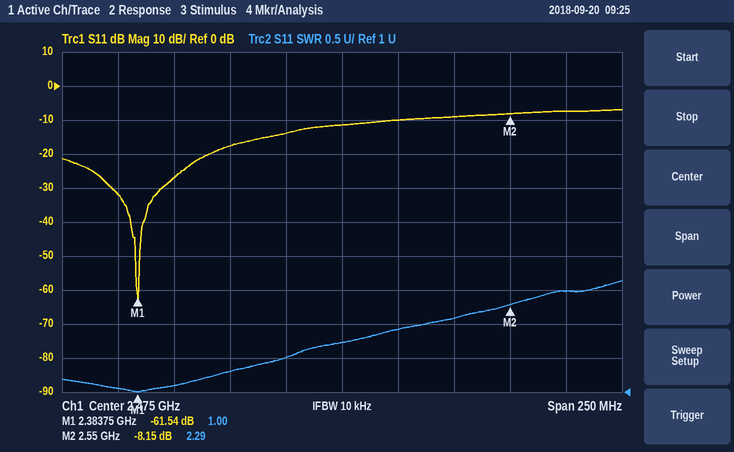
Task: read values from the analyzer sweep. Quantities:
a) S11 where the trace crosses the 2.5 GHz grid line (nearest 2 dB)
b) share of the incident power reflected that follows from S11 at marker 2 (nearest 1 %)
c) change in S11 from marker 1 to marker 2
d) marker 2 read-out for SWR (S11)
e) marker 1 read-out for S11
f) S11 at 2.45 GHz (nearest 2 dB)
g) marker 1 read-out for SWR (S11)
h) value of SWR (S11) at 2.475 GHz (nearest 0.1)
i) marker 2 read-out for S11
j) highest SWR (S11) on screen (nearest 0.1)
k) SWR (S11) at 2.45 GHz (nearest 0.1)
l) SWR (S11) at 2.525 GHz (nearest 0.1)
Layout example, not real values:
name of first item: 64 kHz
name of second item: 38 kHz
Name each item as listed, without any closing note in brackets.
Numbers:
S11 where the trace crosses the 2.5 GHz grid line: -10 dB
share of the incident power reflected that follows from S11 at marker 2: 15 %
change in S11 from marker 1 to marker 2: 53.39 dB
marker 2 read-out for SWR: 2.29
marker 1 read-out for S11: -61.54 dB
S11 at 2.45 GHz: -14 dB
marker 1 read-out for SWR: 1.00
value of SWR (S11) at 2.475 GHz: 1.7
marker 2 read-out for S11: -8.15 dB
highest SWR (S11) on screen: 2.6
SWR (S11) at 2.45 GHz: 1.5
SWR (S11) at 2.525 GHz: 2.1
